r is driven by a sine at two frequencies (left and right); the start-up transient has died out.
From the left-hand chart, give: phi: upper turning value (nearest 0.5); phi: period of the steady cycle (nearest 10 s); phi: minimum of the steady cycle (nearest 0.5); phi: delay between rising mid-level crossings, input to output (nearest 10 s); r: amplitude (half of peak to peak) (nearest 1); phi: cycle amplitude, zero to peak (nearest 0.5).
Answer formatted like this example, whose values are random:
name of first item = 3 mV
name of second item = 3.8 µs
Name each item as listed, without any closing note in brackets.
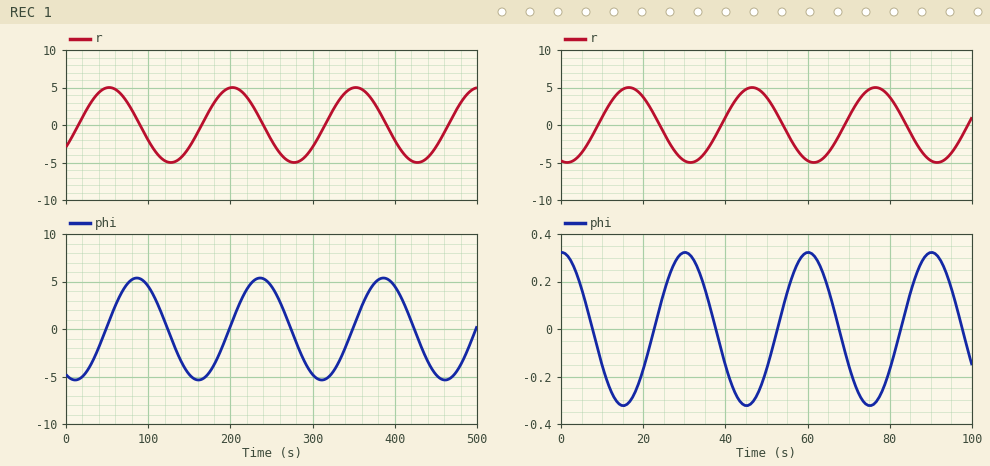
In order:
phi: upper turning value = 5.5
phi: period of the steady cycle = 150 s
phi: minimum of the steady cycle = -5.5
phi: delay between rising mid-level crossings, input to output = 30 s
r: amplitude (half of peak to peak) = 5
phi: cycle amplitude, zero to peak = 5.5
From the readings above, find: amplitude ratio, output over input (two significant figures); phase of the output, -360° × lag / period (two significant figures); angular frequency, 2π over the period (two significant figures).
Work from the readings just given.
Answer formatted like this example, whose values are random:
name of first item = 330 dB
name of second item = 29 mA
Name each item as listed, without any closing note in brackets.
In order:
amplitude ratio, output over input = 1.1
phase of the output, -360° × lag / period = -72°
angular frequency, 2π over the period = 0.042 rad/s
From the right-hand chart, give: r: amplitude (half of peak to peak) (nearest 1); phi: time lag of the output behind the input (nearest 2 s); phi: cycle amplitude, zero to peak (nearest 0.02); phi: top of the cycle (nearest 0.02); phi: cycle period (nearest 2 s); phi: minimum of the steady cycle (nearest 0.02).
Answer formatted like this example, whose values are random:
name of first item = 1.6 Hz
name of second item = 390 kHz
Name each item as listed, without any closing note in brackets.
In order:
r: amplitude (half of peak to peak) = 5
phi: time lag of the output behind the input = 14 s
phi: cycle amplitude, zero to peak = 0.32
phi: top of the cycle = 0.32
phi: cycle period = 30 s
phi: minimum of the steady cycle = -0.32
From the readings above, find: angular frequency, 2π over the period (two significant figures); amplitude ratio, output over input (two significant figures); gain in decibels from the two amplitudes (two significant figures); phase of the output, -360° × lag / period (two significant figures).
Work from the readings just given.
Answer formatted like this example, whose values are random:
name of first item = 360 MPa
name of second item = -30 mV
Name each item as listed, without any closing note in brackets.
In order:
angular frequency, 2π over the period = 0.21 rad/s
amplitude ratio, output over input = 0.064
gain in decibels from the two amplitudes = -24 dB
phase of the output, -360° × lag / period = -170°
